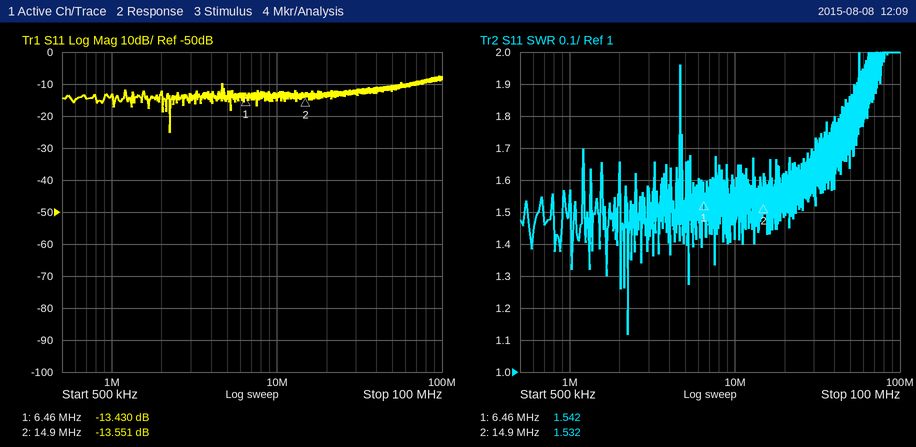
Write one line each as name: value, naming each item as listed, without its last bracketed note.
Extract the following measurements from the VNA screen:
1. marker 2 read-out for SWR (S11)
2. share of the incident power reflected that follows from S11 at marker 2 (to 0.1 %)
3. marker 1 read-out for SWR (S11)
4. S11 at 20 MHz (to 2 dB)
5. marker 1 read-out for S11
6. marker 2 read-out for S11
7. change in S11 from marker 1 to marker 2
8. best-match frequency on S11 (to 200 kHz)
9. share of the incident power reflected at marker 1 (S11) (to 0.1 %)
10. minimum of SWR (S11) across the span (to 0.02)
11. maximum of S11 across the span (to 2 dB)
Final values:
marker 2 read-out for SWR: 1.532
share of the incident power reflected that follows from S11 at marker 2: 4.4 %
marker 1 read-out for SWR: 1.542
S11 at 20 MHz: -14 dB
marker 1 read-out for S11: -13.430 dB
marker 2 read-out for S11: -13.551 dB
change in S11 from marker 1 to marker 2: -0.121 dB
best-match frequency on S11: 2.2 MHz
share of the incident power reflected at marker 1 (S11): 4.5 %
minimum of SWR (S11) across the span: 1.12
maximum of S11 across the span: -8 dB
